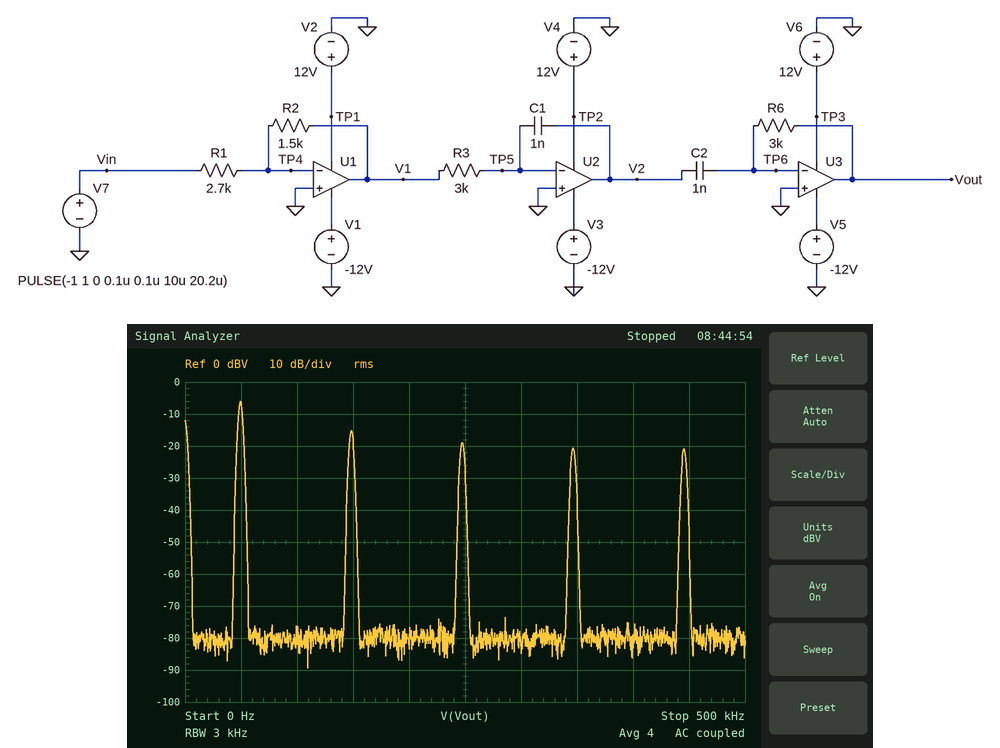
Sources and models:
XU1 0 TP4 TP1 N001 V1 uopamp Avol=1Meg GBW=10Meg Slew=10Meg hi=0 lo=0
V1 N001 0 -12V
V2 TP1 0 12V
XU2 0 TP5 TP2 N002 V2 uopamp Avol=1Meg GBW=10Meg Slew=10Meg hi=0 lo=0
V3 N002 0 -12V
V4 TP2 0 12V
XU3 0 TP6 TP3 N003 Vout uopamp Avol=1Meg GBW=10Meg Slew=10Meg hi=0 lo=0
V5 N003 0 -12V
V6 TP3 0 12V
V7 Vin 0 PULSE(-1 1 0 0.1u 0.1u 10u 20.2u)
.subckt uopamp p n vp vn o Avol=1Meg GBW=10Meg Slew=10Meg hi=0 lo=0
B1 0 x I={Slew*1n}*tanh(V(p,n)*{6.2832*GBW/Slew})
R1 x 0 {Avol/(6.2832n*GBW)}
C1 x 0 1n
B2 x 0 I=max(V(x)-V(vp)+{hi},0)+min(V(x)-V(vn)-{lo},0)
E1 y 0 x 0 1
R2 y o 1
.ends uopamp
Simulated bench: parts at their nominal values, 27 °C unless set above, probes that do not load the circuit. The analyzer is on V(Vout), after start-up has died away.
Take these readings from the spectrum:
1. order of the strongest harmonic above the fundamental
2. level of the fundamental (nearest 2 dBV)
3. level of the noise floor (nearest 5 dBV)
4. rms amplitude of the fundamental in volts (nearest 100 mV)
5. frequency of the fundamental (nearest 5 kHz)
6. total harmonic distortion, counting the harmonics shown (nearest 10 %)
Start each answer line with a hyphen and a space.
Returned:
- 3
- -6 dBV
- -80 dBV
- 500 mV
- 50 kHz
- 50 %
